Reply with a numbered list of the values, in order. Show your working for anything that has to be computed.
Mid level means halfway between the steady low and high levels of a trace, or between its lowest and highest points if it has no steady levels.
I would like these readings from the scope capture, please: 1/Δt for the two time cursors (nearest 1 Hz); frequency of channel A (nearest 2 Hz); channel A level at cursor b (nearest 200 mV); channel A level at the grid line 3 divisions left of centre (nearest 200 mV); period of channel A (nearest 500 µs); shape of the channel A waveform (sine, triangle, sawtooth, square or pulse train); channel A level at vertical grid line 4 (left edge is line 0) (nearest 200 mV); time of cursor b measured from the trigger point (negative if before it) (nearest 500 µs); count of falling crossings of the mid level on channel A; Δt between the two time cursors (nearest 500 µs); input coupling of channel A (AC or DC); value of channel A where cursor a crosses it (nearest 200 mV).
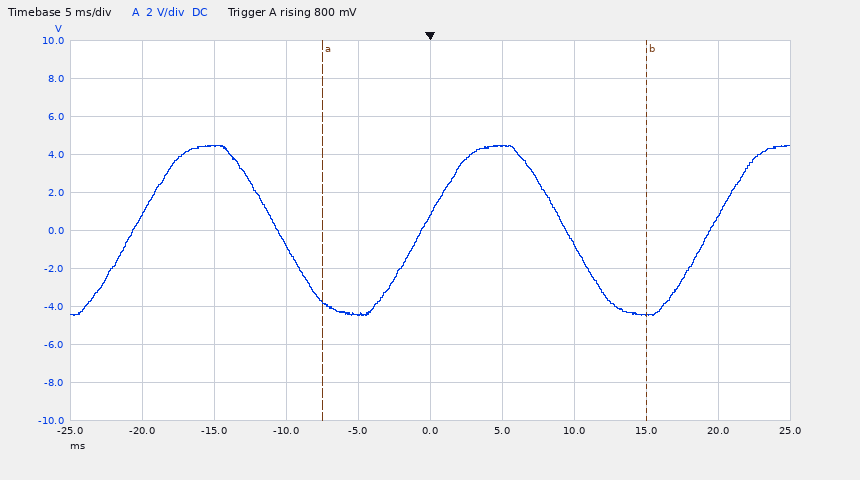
1. 1 / 22.5 ms ≈ 44 Hz
2. 1 / 20.0 ms ≈ 50 Hz
3. -4.4 V
4. 4.4 V
5. 20.0 ms
6. sine
7. -4.4 V
8. +15.0 ms
9. 2
10. 22.5 ms
11. DC
12. -3.8 V
